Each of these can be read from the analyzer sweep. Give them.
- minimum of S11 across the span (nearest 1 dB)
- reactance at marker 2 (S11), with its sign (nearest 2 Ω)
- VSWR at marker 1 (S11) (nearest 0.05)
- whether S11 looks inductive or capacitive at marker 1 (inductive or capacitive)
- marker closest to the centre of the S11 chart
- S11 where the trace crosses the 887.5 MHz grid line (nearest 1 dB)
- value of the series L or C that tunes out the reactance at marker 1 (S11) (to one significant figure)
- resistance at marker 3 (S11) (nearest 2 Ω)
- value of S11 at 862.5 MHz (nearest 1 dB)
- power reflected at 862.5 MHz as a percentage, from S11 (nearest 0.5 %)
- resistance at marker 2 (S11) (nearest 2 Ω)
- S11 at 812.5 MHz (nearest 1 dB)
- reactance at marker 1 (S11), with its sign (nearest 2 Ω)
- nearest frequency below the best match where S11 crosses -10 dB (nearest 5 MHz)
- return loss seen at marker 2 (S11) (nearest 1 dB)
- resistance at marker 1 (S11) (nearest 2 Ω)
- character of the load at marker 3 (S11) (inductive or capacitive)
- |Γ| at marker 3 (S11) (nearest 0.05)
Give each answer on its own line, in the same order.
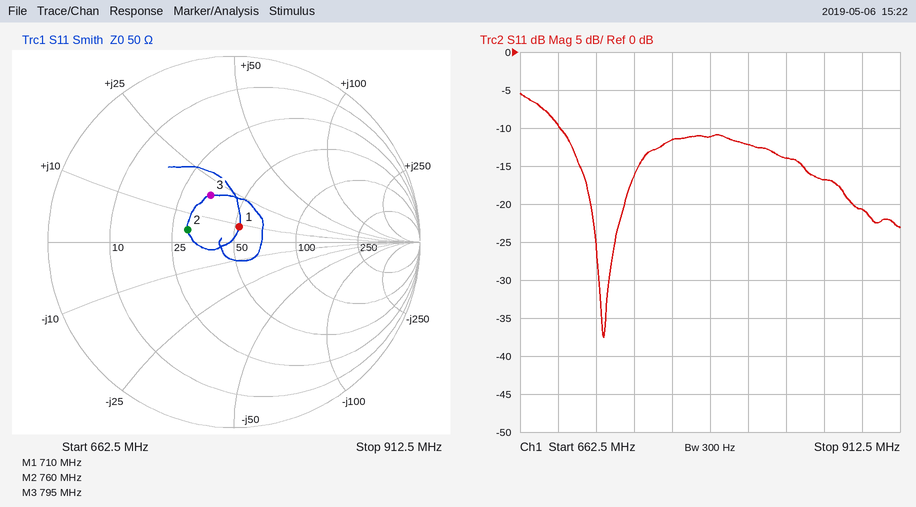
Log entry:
-38 dB
+4 Ω
1.20
inductive
marker 1
-21 dB
30 pF
34 Ω
-17 dB
2.0 %
30 Ω
-12 dB
+8 Ω
690 MHz
12 dB
52 Ω
inductive
0.30
